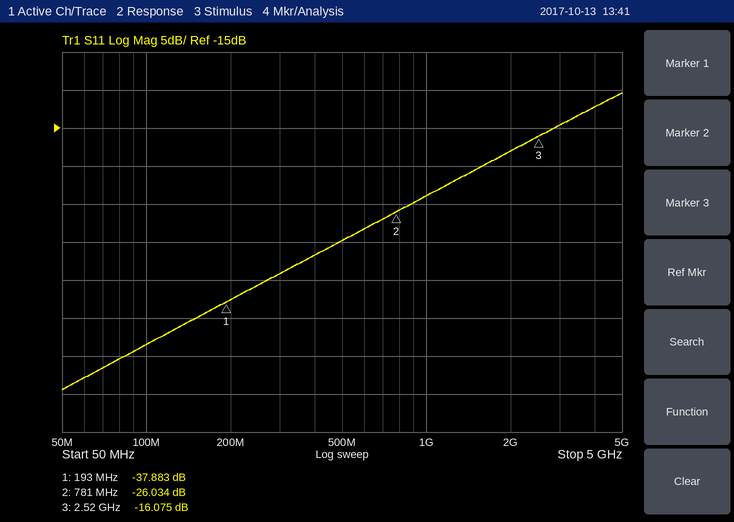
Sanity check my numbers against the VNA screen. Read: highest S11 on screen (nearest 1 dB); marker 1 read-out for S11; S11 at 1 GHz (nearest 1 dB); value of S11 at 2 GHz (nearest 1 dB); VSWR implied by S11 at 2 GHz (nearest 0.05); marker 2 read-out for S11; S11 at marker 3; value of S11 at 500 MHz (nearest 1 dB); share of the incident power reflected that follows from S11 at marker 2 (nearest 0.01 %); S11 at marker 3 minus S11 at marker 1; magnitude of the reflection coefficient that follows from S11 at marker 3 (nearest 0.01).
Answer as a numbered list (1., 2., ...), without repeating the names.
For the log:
1. -10 dB
2. -37.883 dB
3. -24 dB
4. -18 dB
5. 1.30
6. -26.034 dB
7. -16.075 dB
8. -30 dB
9. 0.25 %
10. 21.808 dB
11. 0.16
